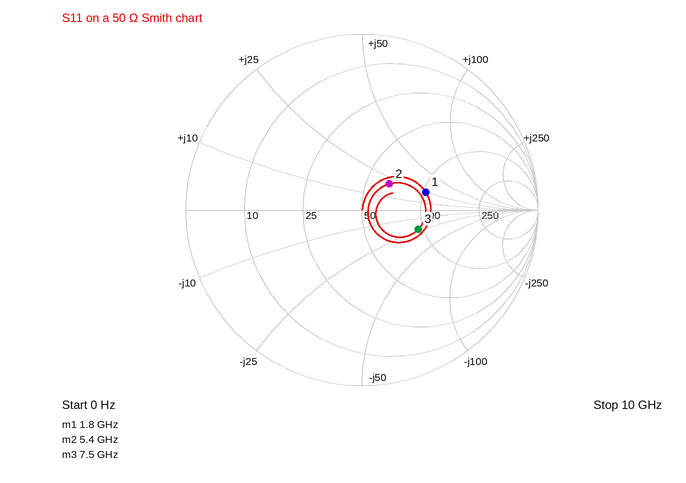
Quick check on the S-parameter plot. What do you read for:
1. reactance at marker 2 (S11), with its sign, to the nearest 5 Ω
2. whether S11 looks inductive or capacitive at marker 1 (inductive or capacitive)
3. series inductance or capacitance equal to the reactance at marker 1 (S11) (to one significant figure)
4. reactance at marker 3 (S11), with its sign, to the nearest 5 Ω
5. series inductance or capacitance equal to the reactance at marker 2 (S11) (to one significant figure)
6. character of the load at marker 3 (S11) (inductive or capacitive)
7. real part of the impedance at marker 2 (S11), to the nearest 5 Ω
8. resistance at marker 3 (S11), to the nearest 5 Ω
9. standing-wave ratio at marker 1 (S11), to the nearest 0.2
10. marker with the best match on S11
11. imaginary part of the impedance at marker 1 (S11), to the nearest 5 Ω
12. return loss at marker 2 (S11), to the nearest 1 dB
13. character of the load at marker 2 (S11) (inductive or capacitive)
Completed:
+20 Ω
inductive
2 nH
-25 Ω
600 pH
capacitive
65 Ω
95 Ω
2.2
marker 2
+25 Ω
13 dB
inductive
